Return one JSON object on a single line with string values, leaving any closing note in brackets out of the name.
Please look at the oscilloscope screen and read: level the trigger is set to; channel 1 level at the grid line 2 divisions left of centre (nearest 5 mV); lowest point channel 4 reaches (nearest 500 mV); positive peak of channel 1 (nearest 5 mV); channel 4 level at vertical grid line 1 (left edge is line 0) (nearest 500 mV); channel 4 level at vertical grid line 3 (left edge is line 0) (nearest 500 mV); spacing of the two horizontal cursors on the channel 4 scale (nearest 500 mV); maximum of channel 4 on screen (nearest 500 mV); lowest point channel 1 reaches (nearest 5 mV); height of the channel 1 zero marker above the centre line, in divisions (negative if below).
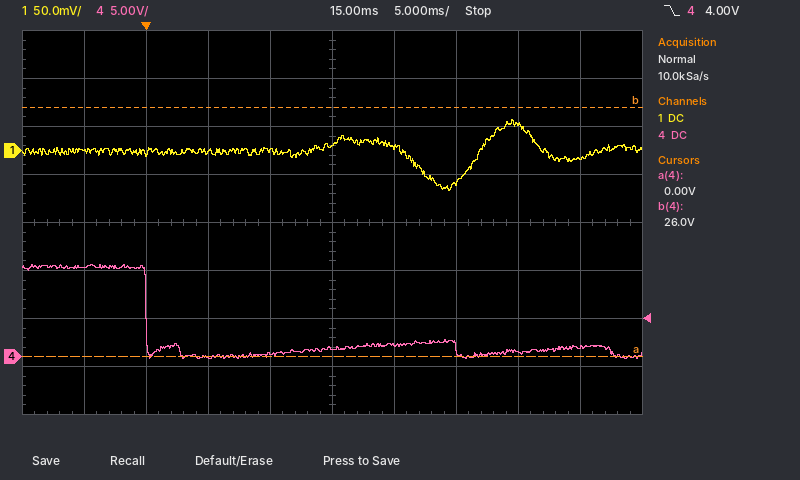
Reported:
{"level the trigger is set to": "4.00 V", "channel 1 level at the grid line 2 divisions left of centre": "0 mV", "lowest point channel 4 reaches": "0.0 V", "positive peak of channel 1": "30 mV", "channel 4 level at vertical grid line 1 (left edge is line 0)": "9.5 V", "channel 4 level at vertical grid line 3 (left edge is line 0)": "0.0 V", "spacing of the two horizontal cursors on the channel 4 scale": "26.0 V", "maximum of channel 4 on screen": "9.5 V", "lowest point channel 1 reaches": "-40 mV", "height of the channel 1 zero marker above the centre line, in divisions": "+1.5 div"}
